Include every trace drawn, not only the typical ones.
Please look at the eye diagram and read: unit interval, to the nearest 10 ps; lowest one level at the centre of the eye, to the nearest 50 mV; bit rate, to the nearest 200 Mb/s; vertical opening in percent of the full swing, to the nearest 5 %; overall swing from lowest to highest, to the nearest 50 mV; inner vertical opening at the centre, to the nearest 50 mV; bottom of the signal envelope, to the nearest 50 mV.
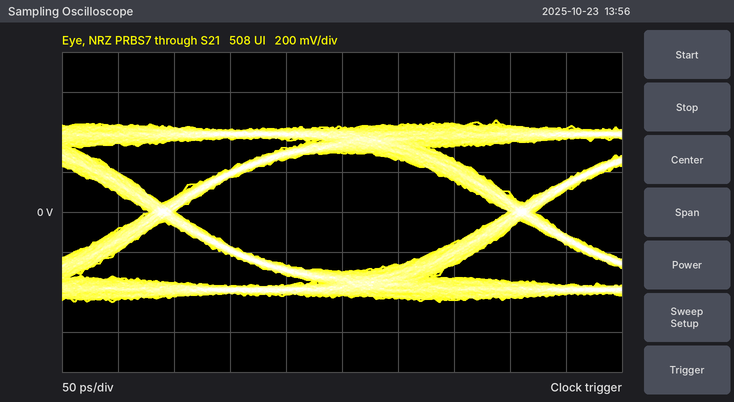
320 ps
300 mV
3.2 Gb/s
65 %
900 mV
600 mV
-450 mV
